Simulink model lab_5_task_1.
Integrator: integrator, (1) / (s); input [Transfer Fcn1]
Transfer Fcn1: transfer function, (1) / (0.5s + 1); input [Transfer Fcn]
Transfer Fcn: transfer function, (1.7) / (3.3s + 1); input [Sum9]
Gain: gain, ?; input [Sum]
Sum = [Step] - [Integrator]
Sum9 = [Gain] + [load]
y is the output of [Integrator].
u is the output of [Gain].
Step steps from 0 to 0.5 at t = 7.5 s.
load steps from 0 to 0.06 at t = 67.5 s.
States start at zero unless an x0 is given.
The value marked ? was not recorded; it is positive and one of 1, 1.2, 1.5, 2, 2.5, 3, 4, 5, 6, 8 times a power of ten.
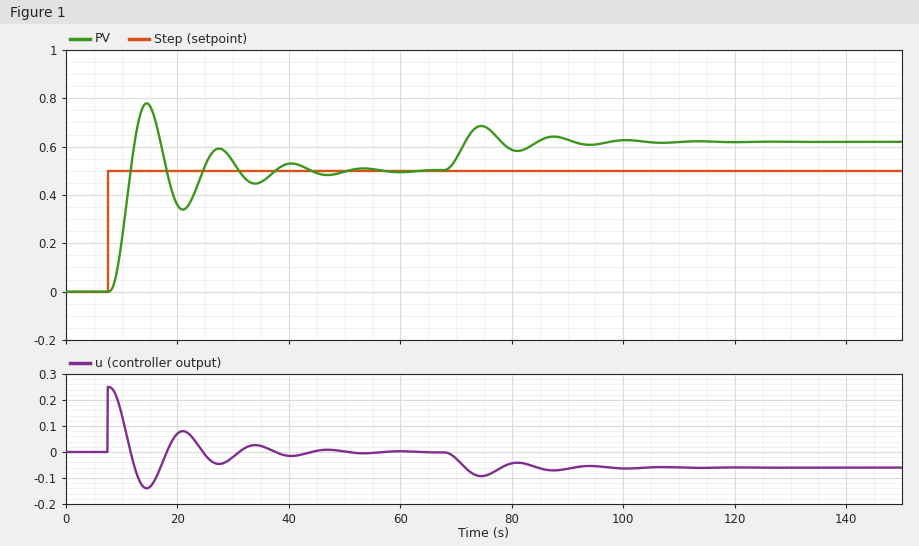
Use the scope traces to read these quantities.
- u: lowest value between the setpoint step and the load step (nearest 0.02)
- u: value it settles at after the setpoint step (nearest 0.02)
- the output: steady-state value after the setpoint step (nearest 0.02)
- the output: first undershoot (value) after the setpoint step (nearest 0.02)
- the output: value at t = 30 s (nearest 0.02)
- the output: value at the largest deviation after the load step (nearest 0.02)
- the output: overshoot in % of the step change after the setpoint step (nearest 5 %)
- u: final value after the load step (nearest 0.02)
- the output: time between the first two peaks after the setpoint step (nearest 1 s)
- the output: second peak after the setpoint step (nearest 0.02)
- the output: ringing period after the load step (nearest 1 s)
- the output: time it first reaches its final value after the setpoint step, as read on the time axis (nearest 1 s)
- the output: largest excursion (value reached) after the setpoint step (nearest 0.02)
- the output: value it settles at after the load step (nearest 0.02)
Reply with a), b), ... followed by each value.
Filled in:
a) -0.14
b) 0.00
c) 0.50
d) 0.34
e) 0.54
f) 0.68
g) 55 %
h) -0.06
i) 13 s
j) 0.60
k) 13 s
l) 12 s
m) 0.78
n) 0.62
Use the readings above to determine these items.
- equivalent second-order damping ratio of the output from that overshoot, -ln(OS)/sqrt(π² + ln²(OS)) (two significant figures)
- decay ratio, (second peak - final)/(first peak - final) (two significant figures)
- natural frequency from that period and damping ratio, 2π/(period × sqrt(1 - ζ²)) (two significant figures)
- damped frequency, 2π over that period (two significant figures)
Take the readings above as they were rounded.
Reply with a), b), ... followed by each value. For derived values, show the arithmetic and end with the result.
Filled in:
a) ln(0.55) = -0.598; 0.598 / sqrt(9.870 + 0.357) = 0.19
b) (0.6 - 0.5) / (0.78 - 0.5) = 0.36
c) 2π / (13 × sqrt(1 - 0.19²)) = 0.49 rad/s
d) 2π / 13 = 0.48 rad/s
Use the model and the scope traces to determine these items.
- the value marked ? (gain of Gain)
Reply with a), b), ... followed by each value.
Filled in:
a) 0.5
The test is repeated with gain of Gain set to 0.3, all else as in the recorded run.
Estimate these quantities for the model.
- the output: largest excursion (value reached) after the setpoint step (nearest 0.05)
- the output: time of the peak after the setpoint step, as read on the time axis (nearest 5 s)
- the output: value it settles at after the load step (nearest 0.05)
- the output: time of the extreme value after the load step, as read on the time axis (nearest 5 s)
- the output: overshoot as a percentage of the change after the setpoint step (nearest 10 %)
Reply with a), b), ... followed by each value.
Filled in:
a) 0.70
b) 15 s
c) 0.70
d) 75 s
e) 40 %
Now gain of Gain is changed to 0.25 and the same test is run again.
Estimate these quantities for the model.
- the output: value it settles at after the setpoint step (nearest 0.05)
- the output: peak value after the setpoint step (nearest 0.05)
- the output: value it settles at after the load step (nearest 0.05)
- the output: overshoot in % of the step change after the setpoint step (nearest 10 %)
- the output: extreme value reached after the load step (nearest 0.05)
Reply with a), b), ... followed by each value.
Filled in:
a) 0.50
b) 0.65
c) 0.75
d) 30 %
e) 0.80
